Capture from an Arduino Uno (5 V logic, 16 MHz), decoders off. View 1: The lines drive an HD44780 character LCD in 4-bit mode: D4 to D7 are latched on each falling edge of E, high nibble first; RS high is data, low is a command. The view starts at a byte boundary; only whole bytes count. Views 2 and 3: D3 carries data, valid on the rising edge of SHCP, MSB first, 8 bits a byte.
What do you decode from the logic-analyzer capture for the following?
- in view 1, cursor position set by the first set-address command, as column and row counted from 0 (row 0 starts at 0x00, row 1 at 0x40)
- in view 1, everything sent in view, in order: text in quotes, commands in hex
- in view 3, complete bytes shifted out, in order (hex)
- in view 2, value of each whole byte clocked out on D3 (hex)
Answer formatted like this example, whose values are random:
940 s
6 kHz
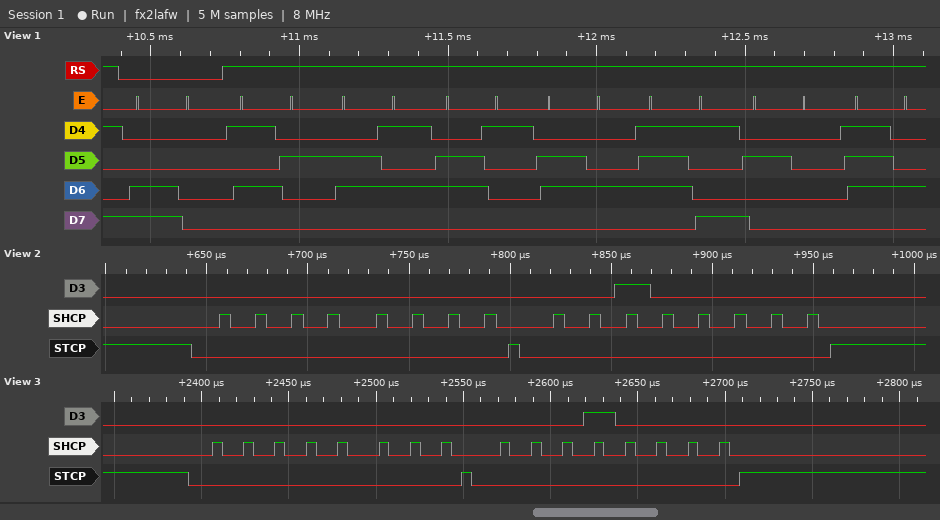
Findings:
column 0, row 1
0xC0 "Ready t"
0x00 0x10
00 20
